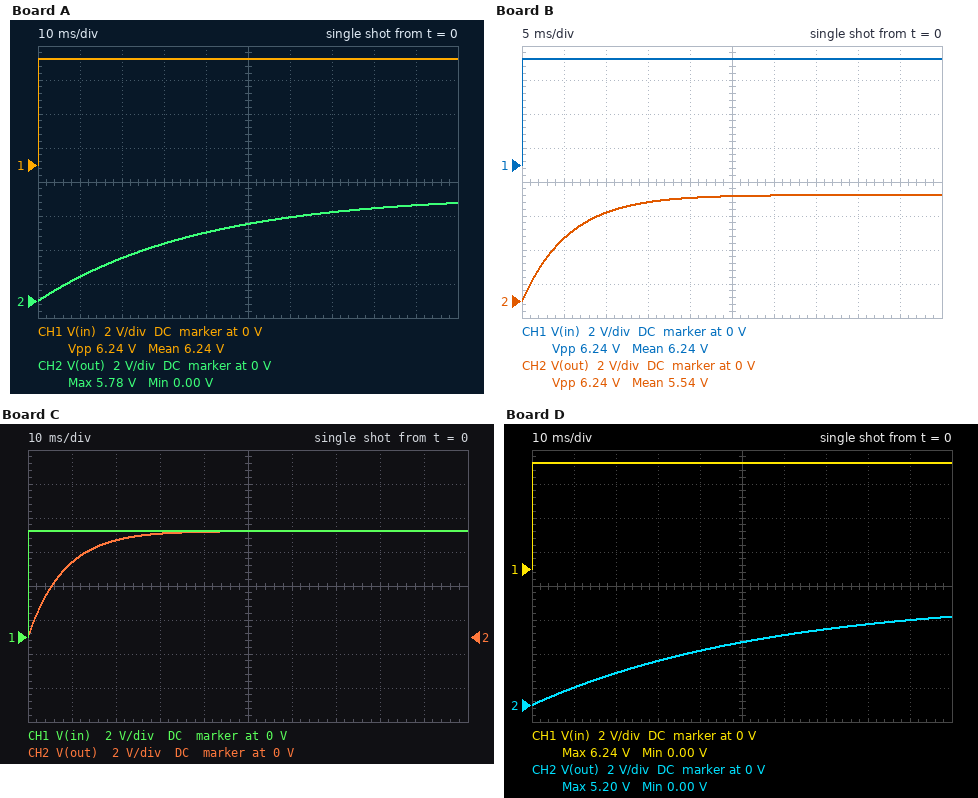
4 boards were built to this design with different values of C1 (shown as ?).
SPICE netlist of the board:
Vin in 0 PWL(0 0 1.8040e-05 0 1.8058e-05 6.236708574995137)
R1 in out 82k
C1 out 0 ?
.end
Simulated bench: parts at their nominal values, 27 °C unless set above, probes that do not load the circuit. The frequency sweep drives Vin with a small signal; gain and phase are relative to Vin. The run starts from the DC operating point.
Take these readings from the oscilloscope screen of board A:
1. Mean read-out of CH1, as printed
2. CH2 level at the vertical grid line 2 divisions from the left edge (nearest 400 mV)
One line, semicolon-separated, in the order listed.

6.24 V; 2.4 V
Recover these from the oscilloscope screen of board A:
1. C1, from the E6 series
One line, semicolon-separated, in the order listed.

470 nF
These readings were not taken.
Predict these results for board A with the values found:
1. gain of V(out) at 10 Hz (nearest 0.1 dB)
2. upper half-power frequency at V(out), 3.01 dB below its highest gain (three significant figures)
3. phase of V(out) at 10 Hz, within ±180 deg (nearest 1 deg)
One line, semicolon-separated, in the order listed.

-8.4 dB; 4.13 Hz; -68 deg
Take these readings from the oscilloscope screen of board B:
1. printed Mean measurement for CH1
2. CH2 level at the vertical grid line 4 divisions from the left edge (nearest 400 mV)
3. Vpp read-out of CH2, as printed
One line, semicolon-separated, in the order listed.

6.24 V; 6.0 V; 6.24 V
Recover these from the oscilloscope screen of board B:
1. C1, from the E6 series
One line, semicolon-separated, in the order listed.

68 nF
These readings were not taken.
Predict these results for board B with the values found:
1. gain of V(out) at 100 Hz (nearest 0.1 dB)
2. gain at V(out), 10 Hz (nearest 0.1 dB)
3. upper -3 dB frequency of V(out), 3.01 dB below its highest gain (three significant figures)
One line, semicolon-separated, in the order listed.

-11.2 dB; -0.5 dB; 28.5 Hz
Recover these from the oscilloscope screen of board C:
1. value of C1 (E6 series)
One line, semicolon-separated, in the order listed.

100 nF
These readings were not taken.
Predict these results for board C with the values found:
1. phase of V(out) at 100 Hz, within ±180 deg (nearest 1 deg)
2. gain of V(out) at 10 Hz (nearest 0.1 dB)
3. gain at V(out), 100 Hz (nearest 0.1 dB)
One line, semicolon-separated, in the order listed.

-79 deg; -1.0 dB; -14.4 dB
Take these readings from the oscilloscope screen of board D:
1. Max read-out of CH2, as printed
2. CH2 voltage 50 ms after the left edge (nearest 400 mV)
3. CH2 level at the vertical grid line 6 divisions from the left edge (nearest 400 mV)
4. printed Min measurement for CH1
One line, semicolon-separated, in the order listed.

5.20 V; 3.6 V; 4.0 V; 0.00 V
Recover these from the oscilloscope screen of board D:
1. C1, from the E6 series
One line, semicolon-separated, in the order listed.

680 nF
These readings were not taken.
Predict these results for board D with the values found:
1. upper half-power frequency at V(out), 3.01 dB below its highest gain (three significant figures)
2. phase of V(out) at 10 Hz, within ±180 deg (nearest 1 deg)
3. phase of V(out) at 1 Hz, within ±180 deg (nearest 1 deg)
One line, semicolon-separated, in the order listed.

2.85 Hz; -74 deg; -19 deg
